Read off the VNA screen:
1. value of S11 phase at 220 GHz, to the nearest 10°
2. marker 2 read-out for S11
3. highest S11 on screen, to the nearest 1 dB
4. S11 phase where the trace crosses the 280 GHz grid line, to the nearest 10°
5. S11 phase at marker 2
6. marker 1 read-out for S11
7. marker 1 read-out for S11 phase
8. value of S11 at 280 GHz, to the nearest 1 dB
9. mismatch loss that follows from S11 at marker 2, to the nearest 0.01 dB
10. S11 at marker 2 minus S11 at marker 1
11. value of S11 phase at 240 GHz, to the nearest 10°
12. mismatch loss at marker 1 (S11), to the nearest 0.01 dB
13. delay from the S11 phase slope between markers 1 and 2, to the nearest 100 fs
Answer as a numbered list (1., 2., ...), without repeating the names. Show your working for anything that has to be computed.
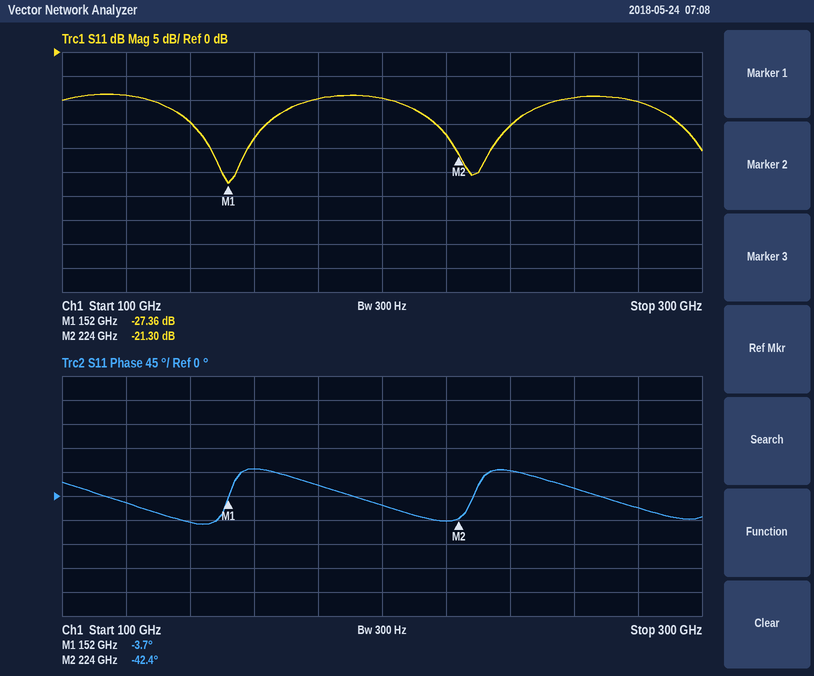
1. -50°
2. -21.30 dB
3. -9 dB
4. -20°
5. -42.4°
6. -27.36 dB
7. -3.7°
8. -10 dB
9. −10 log10(1 − 10^(-21.3/10)) ≈ 0.03 dB
10. -21.3 − (-27.36) = 6.06 dB
11. 50°
12. −10 log10(1 − 10^(-27.36/10)) ≈ 0.01 dB
13. −(-42.4° − (-3.7°))/(360° × 72 GHz) ≈ 1.5 ps
